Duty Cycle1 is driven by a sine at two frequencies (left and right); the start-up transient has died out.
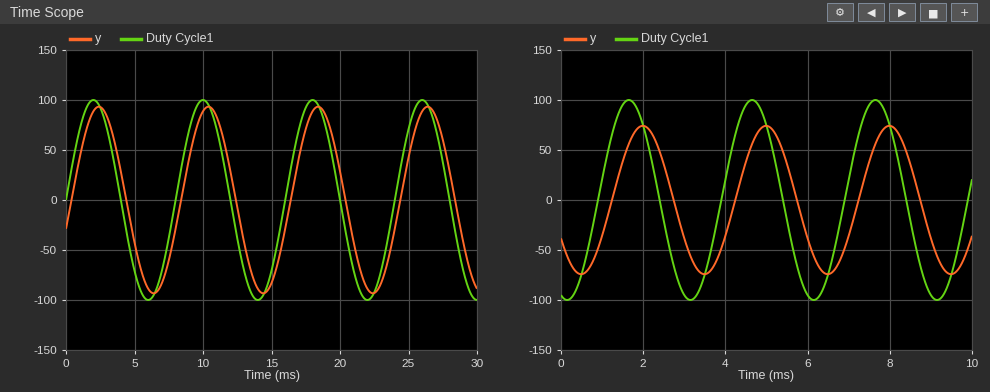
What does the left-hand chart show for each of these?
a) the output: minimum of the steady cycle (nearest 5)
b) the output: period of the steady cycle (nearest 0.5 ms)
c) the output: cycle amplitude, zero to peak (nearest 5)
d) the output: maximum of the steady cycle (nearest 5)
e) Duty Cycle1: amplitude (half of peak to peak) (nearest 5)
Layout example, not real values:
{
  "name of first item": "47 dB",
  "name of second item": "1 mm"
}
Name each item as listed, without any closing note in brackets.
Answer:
{
  "the output: minimum of the steady cycle": "-95",
  "the output: period of the steady cycle": "8.0 ms",
  "the output: cycle amplitude, zero to peak": "95",
  "the output: maximum of the steady cycle": "95",
  "Duty Cycle1: amplitude (half of peak to peak)": "100"
}
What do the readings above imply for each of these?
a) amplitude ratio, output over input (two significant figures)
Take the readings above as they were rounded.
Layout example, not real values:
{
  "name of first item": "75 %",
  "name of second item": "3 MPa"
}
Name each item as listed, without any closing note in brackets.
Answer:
{
  "amplitude ratio, output over input": "0.95"
}
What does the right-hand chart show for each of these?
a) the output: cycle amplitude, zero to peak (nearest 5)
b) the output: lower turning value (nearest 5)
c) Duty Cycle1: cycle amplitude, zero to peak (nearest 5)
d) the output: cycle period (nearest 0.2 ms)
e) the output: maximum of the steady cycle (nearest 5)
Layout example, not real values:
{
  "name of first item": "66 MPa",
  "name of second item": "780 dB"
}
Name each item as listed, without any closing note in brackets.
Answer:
{
  "the output: cycle amplitude, zero to peak": "75",
  "the output: lower turning value": "-75",
  "Duty Cycle1: cycle amplitude, zero to peak": "100",
  "the output: cycle period": "3.0 ms",
  "the output: maximum of the steady cycle": "75"
}
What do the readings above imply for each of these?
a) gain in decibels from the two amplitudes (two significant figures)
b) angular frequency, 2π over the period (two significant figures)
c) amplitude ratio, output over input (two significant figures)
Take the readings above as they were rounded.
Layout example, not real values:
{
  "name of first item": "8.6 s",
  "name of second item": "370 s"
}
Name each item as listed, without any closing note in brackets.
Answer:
{
  "gain in decibels from the two amplitudes": "-2.5 dB",
  "angular frequency, 2π over the period": "2.1 rad/ms",
  "amplitude ratio, output over input": "0.75"
}
